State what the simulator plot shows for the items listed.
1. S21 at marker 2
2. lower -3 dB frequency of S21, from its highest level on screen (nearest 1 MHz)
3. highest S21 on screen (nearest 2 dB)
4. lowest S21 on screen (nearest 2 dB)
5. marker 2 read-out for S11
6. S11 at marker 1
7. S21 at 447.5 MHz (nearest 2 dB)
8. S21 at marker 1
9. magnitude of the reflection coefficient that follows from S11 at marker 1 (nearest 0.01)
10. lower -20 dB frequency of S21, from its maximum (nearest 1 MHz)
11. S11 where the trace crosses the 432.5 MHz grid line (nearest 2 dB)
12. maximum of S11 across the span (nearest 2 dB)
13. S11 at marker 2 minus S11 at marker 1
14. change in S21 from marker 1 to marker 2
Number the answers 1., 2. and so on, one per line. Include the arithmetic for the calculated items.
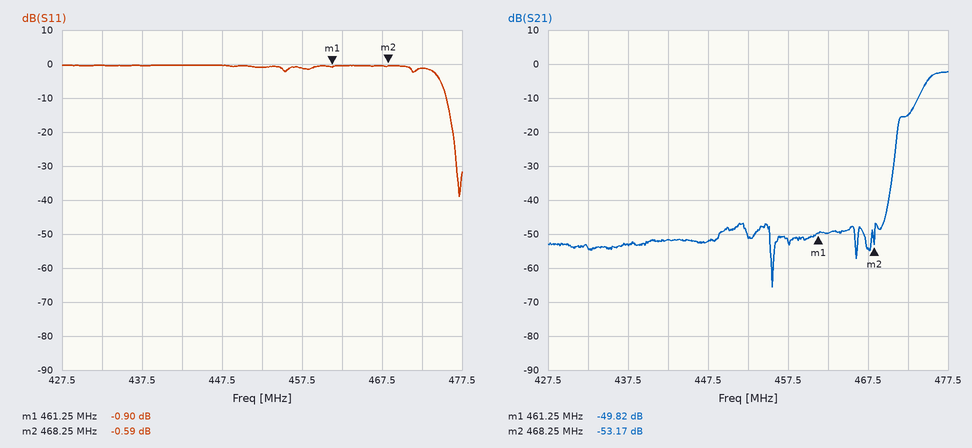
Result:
1. -53.17 dB
2. 475 MHz
3. -2 dB
4. -66 dB
5. -0.59 dB
6. -0.90 dB
7. -52 dB
8. -49.82 dB
9. 10^(-0.9/20) ≈ 0.90
10. 471 MHz
11. 0 dB
12. 0 dB
13. -0.59 − (-0.9) = 0.31 dB
14. -53.17 − (-49.82) = -3.35 dB
